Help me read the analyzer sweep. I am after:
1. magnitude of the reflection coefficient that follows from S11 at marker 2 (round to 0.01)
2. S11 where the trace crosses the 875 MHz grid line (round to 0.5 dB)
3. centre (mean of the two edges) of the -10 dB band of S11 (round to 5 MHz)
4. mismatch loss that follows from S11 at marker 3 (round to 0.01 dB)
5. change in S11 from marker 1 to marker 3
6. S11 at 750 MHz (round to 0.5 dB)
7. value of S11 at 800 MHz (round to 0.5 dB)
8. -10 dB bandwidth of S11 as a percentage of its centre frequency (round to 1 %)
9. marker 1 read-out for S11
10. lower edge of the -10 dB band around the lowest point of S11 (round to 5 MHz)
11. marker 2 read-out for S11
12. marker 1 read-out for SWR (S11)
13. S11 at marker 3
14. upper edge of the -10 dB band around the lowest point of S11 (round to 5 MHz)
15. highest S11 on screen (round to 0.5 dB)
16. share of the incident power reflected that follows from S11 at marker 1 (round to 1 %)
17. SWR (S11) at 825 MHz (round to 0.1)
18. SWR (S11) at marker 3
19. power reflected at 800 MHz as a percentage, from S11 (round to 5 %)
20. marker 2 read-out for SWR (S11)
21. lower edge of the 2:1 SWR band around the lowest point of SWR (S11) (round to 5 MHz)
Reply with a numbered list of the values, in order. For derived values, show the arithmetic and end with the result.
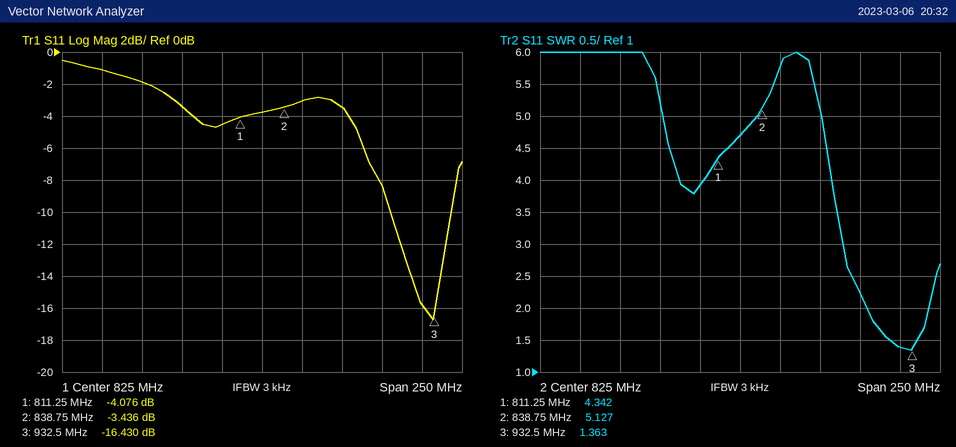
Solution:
1. 10^(-3.436/20) ≈ 0.67
2. -3.5 dB
3. 925 MHz
4. −10 log10(1 − 10^(-16.43/10)) ≈ 0.10 dB
5. -16.43 − (-4.076) = -12.354 dB
6. -2.0 dB
7. -4.5 dB
8. 40 MHz / 925 MHz ≈ 4 %
9. -4.076 dB
10. 905 MHz
11. -3.436 dB
12. 4.342
13. -16.430 dB
14. 945 MHz
15. -0.5 dB
16. 10^(-4.076/10) ≈ 39 %
17. 4.7
18. 1.363
19. 10^(-4.5/10) ≈ 35 %
20. 5.127
21. 905 MHz
